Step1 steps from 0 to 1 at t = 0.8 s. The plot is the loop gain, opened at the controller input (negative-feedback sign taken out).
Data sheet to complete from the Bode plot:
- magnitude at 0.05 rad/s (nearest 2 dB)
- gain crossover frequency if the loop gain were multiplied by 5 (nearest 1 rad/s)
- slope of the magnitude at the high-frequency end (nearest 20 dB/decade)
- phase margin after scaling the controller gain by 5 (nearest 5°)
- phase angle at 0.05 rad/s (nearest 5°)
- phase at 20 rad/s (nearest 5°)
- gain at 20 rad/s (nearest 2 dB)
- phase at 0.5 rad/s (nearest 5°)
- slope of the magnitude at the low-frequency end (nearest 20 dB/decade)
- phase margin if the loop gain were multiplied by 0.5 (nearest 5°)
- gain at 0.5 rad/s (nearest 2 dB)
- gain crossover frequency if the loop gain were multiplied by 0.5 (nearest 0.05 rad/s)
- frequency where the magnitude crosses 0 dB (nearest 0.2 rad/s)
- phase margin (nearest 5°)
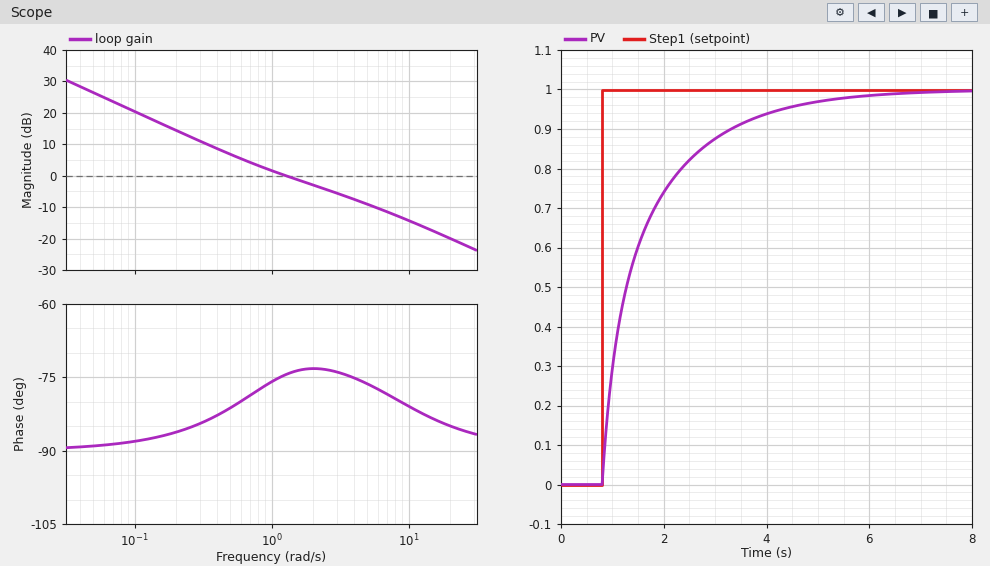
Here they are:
26 dB
10 rad/s
-20 dB/decade
100°
-90°
-85°
-20 dB
-80°
-20 dB/decade
100°
6 dB
0.55 rad/s
1.2 rad/s
105°
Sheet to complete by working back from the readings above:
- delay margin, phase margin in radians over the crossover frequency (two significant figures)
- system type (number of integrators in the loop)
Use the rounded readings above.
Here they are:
1.5 s
1
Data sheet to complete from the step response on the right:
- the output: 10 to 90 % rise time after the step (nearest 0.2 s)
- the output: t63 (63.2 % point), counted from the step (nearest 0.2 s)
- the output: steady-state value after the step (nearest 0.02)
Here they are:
2.4 s
0.8 s
1.00
